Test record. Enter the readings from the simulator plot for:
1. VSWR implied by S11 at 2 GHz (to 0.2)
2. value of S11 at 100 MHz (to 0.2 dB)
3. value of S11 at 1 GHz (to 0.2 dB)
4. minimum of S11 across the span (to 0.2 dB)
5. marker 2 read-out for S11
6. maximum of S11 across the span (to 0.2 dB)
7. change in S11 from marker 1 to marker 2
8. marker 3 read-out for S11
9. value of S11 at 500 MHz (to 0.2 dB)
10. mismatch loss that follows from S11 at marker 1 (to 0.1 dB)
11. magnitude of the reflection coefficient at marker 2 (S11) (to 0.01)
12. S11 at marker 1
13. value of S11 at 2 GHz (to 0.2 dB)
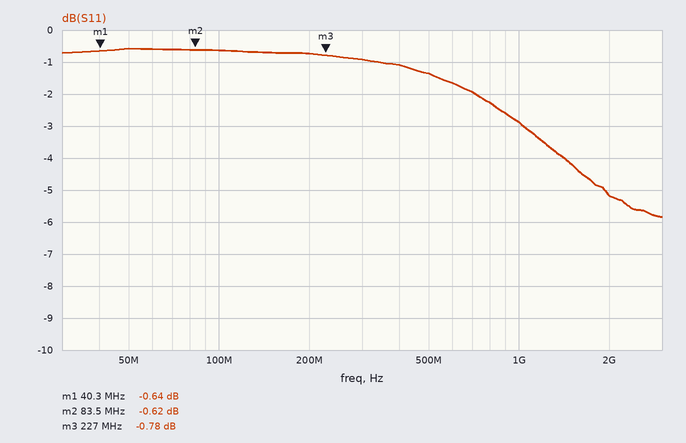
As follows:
3.4
-0.6 dB
-2.8 dB
-5.8 dB
-0.62 dB
-0.6 dB
0.02 dB
-0.78 dB
-1.4 dB
8.6 dB
0.93
-0.64 dB
-5.2 dB
